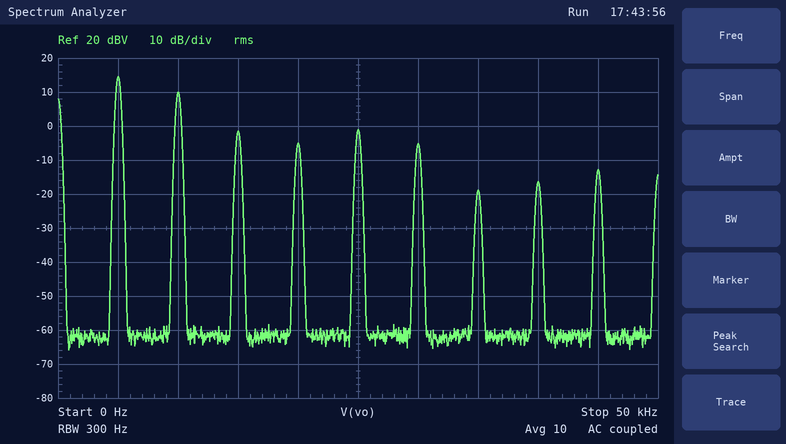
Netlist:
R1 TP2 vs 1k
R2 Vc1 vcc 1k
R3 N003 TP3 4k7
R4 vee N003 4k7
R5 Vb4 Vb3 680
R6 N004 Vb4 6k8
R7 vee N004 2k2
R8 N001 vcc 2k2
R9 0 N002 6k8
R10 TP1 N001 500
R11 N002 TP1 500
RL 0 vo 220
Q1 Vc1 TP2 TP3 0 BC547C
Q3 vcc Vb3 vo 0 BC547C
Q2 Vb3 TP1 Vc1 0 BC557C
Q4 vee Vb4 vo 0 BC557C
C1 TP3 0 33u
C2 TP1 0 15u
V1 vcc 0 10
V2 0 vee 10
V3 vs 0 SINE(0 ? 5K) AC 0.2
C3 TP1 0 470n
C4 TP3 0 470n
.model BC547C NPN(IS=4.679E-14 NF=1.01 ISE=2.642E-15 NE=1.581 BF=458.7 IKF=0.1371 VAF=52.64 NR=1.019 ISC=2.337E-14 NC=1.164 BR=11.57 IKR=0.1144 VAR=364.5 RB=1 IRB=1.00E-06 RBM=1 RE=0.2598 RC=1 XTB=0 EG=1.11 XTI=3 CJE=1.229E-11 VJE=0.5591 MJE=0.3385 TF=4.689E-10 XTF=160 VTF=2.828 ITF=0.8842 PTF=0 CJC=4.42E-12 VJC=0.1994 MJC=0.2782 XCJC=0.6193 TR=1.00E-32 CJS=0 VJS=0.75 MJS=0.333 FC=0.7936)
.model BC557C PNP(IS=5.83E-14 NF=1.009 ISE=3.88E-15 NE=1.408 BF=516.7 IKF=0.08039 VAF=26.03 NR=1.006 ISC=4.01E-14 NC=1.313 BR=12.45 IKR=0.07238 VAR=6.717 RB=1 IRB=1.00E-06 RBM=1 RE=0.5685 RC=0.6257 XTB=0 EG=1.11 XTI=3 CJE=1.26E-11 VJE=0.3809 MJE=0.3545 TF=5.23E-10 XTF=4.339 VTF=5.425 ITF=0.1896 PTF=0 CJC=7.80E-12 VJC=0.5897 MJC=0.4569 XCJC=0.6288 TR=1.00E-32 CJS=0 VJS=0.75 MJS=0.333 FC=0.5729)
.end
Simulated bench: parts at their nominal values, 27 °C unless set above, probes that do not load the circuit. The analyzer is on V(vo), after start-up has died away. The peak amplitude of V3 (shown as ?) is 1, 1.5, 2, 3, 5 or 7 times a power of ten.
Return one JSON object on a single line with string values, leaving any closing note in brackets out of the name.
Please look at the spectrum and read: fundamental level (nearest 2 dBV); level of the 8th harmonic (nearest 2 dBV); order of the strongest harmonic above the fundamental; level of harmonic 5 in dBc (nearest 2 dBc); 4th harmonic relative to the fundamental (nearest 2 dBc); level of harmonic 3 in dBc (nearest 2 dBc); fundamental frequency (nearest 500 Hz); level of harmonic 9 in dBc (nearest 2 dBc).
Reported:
{"fundamental level": "14 dBV", "level of the 8th harmonic": "-16 dBV", "order of the strongest harmonic above the fundamental": "2", "level of harmonic 5 in dBc": "-16 dBc", "4th harmonic relative to the fundamental": "-20 dBc", "level of harmonic 3 in dBc": "-16 dBc", "fundamental frequency": "5.0 kHz", "level of harmonic 9 in dBc": "-28 dBc"}
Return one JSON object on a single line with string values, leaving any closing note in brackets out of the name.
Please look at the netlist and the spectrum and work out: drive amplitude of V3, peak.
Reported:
{"drive amplitude of V3, peak": "150 mV"}
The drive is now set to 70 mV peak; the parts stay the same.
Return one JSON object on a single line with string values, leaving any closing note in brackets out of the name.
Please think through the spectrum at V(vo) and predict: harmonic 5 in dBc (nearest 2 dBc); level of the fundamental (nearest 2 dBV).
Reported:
{"harmonic 5 in dBc": "-24 dBc", "level of the fundamental": "16 dBV"}
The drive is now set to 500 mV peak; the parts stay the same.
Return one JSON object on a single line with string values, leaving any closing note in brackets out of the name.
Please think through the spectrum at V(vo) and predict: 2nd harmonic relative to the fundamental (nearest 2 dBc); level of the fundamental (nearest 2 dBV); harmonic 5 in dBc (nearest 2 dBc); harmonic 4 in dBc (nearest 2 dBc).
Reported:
{"2nd harmonic relative to the fundamental": "-2 dBc", "level of the fundamental": "12 dBV", "harmonic 5 in dBc": "-24 dBc", "harmonic 4 in dBc": "-10 dBc"}
